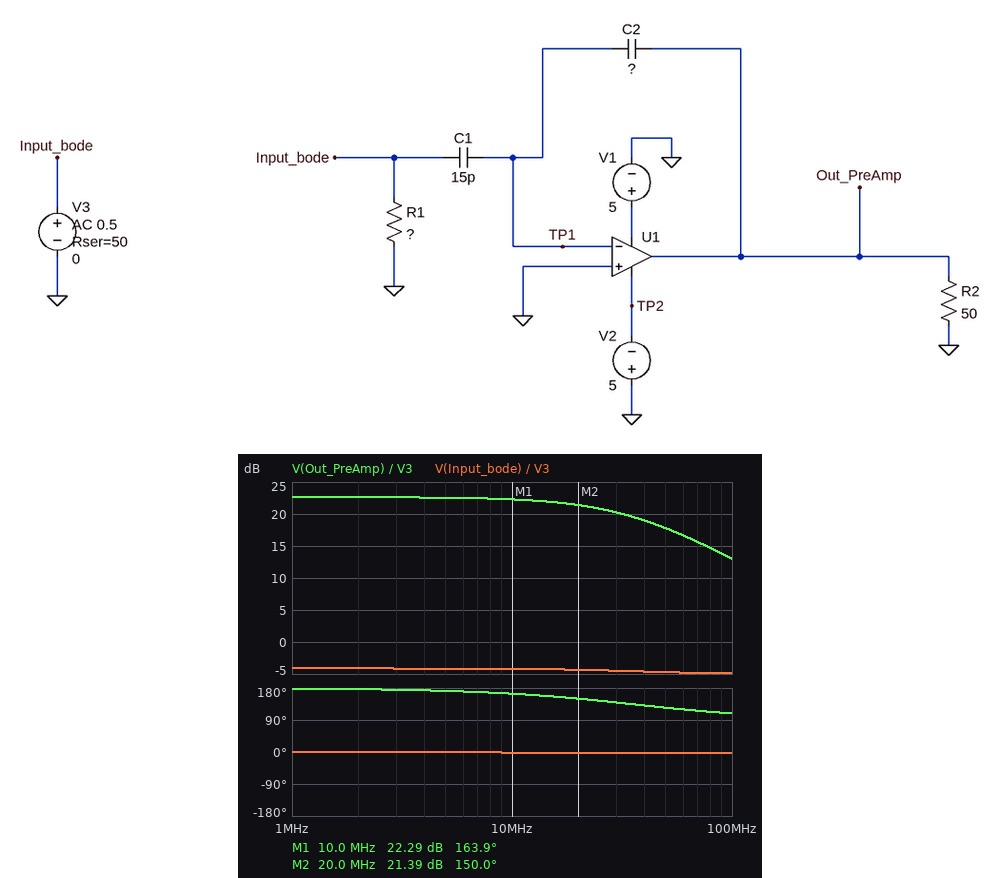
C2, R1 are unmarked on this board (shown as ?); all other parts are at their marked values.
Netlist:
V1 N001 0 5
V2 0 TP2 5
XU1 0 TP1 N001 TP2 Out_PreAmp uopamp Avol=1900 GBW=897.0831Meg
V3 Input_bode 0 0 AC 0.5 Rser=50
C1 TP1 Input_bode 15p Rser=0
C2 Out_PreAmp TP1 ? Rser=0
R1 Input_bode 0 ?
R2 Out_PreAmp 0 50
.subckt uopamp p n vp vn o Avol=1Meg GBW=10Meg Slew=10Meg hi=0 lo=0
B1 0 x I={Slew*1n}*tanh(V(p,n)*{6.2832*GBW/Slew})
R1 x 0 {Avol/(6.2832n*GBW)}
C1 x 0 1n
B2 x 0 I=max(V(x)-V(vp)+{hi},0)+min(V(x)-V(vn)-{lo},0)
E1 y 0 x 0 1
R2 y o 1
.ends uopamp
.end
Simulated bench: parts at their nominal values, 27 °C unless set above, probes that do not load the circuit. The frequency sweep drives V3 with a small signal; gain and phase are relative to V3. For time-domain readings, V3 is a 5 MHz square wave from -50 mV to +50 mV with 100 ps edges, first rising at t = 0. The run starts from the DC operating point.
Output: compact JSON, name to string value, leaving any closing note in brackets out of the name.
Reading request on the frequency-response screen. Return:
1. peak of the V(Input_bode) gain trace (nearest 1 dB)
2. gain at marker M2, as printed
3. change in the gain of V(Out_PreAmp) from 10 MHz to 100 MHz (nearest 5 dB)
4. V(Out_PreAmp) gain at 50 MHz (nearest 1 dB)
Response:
{"peak of the V(Input_bode) gain trace": "-4 dB", "gain at marker M2, as printed": "21.39 dB", "change in the gain of V(Out_PreAmp) from 10 MHz to 100 MHz": "-10 dB", "V(Out_PreAmp) gain at 50 MHz": "18 dB"}
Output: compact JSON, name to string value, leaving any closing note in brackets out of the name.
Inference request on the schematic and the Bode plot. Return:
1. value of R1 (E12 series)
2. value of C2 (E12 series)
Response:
{"value of R1": "82 Ω", "value of C2": "680 fF"}
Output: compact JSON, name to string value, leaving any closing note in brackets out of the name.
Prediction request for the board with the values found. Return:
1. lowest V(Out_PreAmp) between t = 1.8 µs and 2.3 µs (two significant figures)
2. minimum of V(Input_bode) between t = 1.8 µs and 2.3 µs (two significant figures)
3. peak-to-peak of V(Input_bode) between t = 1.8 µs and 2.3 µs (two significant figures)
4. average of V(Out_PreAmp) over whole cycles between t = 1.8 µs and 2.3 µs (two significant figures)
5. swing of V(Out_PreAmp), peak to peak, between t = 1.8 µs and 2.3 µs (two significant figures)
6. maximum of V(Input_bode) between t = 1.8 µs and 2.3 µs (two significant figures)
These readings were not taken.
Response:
{"lowest V(Out_PreAmp) between t = 1.8 µs and 2.3 µs": "-850 mV", "minimum of V(Input_bode) between t = 1.8 µs and 2.3 µs": "-31 mV", "peak-to-peak of V(Input_bode) between t = 1.8 µs and 2.3 µs": "62 mV", "average of V(Out_PreAmp) over whole cycles between t = 1.8 µs and 2.3 µs": "-380 mV", "swing of V(Out_PreAmp), peak to peak, between t = 1.8 µs and 2.3 µs": "850 mV", "maximum of V(Input_bode) between t = 1.8 µs and 2.3 µs": "31 mV"}
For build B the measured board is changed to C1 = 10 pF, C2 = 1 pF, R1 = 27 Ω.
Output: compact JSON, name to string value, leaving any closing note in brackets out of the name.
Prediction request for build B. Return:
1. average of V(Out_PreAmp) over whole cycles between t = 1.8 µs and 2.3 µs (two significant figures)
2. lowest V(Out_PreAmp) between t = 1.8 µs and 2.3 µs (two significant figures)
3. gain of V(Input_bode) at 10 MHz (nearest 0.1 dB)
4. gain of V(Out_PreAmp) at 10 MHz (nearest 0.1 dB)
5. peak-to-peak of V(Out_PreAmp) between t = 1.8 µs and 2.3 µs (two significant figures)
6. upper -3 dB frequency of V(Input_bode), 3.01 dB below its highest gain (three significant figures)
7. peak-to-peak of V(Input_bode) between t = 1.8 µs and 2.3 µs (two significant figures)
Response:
{"average of V(Out_PreAmp) over whole cycles between t = 1.8 µs and 2.3 µs": "-170 mV", "lowest V(Out_PreAmp) between t = 1.8 µs and 2.3 µs": "-350 mV", "gain of V(Input_bode) at 10 MHz": "-9.1 dB", "gain of V(Out_PreAmp) at 10 MHz": "10.8 dB", "peak-to-peak of V(Out_PreAmp) between t = 1.8 µs and 2.3 µs": "350 mV", "upper -3 dB frequency of V(Input_bode), 3.01 dB below its highest gain": "8.65 GHz", "peak-to-peak of V(Input_bode) between t = 1.8 µs and 2.3 µs": "35 mV"}
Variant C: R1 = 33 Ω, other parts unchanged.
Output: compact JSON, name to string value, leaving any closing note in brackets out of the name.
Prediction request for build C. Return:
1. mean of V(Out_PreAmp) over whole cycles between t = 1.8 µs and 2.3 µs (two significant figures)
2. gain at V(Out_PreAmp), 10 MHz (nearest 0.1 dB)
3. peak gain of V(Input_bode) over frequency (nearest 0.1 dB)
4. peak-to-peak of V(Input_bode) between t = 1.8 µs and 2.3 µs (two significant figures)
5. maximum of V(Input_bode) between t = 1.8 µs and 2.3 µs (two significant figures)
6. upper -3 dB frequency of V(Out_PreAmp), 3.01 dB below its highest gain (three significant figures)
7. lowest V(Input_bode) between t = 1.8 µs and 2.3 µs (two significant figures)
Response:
{"mean of V(Out_PreAmp) over whole cycles between t = 1.8 µs and 2.3 µs": "-380 mV", "gain at V(Out_PreAmp), 10 MHz": "18.4 dB", "peak gain of V(Input_bode) over frequency": "-8.0 dB", "peak-to-peak of V(Input_bode) between t = 1.8 µs and 2.3 µs": "40 mV", "maximum of V(Input_bode) between t = 1.8 µs and 2.3 µs": "20 mV", "upper -3 dB frequency of V(Out_PreAmp), 3.01 dB below its highest gain": "36.1 MHz", "lowest V(Input_bode) between t = 1.8 µs and 2.3 µs": "-20 mV"}
